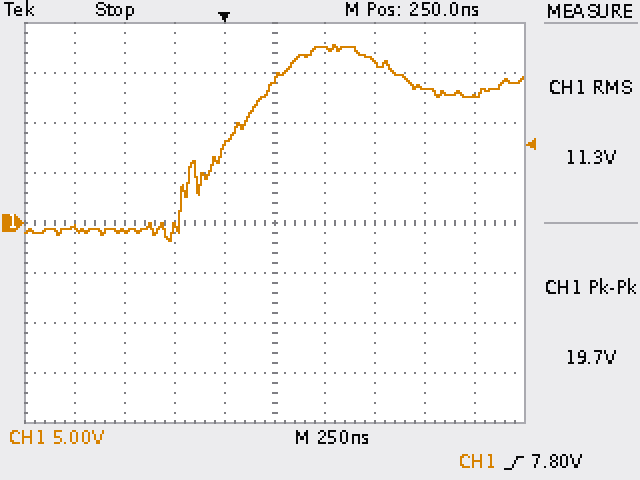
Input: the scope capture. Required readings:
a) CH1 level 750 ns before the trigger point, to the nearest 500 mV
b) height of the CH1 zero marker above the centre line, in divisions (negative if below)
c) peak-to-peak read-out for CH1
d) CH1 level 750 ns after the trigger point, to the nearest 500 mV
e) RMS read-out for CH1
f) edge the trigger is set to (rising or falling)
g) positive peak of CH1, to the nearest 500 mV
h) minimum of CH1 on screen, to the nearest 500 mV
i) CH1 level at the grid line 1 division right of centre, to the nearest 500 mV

-500 mV
0.0 div
19.7 V
16.0 V
11.3 V
rising
18.0 V
-2.0 V
17.5 V
